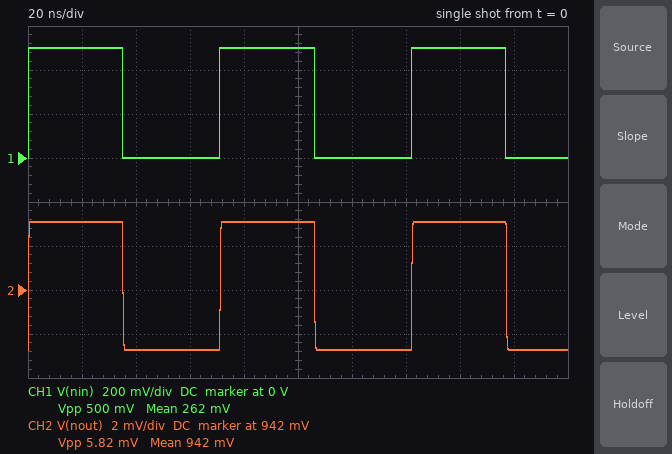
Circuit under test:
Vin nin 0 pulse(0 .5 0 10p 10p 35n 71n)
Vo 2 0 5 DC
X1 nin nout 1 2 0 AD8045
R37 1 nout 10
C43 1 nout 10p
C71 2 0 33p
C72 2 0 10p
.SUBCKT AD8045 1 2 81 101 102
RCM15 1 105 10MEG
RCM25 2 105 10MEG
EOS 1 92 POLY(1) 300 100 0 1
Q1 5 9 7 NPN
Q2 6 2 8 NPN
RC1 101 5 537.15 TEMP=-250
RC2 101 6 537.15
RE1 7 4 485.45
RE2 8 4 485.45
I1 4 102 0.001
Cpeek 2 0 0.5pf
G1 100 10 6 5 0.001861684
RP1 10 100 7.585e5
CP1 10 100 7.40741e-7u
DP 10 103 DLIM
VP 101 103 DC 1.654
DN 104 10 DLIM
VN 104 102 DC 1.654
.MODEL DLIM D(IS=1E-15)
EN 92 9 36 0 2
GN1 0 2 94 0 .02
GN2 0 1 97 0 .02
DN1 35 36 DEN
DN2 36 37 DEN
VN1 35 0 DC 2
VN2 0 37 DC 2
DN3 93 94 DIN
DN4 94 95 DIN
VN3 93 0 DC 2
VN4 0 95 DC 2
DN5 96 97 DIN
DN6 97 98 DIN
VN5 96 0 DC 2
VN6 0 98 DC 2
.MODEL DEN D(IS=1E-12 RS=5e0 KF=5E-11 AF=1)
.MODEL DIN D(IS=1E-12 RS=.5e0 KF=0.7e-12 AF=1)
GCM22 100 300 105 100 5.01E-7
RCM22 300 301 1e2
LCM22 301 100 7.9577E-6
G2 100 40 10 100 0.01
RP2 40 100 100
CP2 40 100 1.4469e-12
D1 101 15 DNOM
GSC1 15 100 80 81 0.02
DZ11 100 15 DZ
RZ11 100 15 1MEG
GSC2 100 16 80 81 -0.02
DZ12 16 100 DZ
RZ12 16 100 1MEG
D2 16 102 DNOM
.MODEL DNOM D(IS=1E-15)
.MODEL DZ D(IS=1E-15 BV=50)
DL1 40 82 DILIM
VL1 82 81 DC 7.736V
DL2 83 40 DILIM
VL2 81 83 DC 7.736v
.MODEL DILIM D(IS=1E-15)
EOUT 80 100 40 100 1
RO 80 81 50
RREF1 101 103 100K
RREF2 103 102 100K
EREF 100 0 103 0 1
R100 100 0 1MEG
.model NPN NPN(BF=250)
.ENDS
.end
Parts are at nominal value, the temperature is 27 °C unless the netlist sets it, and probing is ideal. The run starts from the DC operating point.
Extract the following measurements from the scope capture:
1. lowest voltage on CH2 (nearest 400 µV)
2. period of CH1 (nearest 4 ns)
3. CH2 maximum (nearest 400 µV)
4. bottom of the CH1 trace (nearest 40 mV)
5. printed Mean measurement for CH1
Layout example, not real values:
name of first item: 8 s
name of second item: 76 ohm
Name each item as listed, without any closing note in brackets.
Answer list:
lowest voltage on CH2: 939.2 mV
period of CH1: 72 ns
CH2 maximum: 945.2 mV
bottom of the CH1 trace: 0 V
printed Mean measurement for CH1: 262 mV
